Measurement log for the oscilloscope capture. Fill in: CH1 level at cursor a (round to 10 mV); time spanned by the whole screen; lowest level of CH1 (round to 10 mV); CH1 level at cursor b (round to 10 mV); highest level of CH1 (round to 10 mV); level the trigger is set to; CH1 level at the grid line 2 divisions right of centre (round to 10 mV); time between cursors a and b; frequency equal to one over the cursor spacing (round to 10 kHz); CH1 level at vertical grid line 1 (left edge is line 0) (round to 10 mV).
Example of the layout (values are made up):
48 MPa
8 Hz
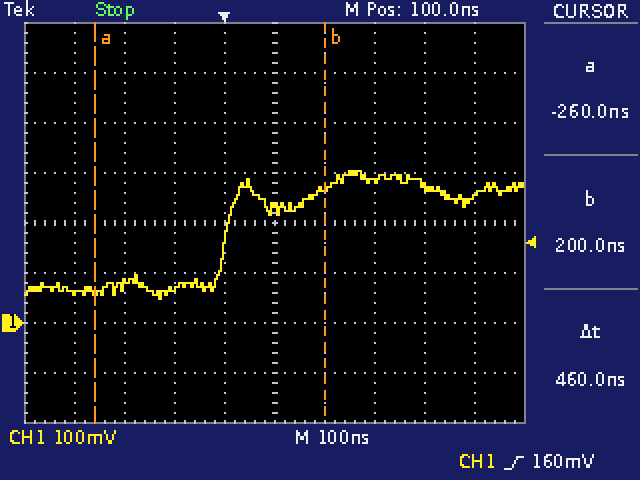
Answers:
60 mV
1 µs
50 mV
270 mV
300 mV
160 mV
280 mV
460 ns
2.17 MHz
60 mV
